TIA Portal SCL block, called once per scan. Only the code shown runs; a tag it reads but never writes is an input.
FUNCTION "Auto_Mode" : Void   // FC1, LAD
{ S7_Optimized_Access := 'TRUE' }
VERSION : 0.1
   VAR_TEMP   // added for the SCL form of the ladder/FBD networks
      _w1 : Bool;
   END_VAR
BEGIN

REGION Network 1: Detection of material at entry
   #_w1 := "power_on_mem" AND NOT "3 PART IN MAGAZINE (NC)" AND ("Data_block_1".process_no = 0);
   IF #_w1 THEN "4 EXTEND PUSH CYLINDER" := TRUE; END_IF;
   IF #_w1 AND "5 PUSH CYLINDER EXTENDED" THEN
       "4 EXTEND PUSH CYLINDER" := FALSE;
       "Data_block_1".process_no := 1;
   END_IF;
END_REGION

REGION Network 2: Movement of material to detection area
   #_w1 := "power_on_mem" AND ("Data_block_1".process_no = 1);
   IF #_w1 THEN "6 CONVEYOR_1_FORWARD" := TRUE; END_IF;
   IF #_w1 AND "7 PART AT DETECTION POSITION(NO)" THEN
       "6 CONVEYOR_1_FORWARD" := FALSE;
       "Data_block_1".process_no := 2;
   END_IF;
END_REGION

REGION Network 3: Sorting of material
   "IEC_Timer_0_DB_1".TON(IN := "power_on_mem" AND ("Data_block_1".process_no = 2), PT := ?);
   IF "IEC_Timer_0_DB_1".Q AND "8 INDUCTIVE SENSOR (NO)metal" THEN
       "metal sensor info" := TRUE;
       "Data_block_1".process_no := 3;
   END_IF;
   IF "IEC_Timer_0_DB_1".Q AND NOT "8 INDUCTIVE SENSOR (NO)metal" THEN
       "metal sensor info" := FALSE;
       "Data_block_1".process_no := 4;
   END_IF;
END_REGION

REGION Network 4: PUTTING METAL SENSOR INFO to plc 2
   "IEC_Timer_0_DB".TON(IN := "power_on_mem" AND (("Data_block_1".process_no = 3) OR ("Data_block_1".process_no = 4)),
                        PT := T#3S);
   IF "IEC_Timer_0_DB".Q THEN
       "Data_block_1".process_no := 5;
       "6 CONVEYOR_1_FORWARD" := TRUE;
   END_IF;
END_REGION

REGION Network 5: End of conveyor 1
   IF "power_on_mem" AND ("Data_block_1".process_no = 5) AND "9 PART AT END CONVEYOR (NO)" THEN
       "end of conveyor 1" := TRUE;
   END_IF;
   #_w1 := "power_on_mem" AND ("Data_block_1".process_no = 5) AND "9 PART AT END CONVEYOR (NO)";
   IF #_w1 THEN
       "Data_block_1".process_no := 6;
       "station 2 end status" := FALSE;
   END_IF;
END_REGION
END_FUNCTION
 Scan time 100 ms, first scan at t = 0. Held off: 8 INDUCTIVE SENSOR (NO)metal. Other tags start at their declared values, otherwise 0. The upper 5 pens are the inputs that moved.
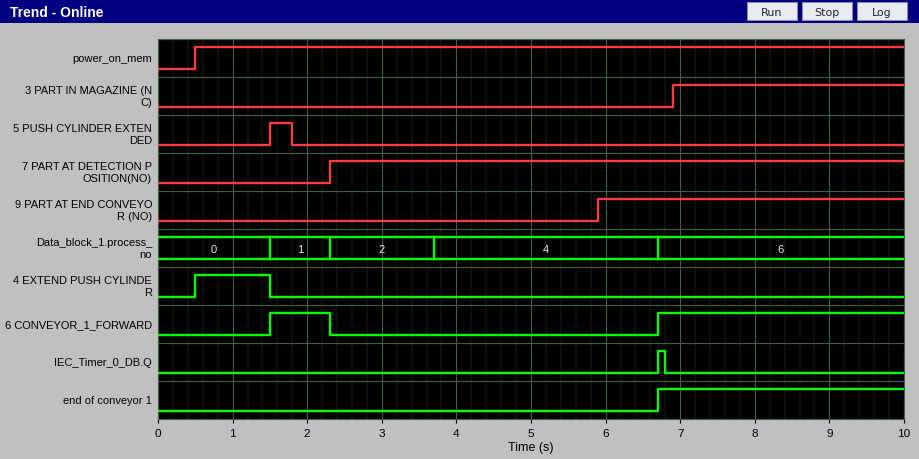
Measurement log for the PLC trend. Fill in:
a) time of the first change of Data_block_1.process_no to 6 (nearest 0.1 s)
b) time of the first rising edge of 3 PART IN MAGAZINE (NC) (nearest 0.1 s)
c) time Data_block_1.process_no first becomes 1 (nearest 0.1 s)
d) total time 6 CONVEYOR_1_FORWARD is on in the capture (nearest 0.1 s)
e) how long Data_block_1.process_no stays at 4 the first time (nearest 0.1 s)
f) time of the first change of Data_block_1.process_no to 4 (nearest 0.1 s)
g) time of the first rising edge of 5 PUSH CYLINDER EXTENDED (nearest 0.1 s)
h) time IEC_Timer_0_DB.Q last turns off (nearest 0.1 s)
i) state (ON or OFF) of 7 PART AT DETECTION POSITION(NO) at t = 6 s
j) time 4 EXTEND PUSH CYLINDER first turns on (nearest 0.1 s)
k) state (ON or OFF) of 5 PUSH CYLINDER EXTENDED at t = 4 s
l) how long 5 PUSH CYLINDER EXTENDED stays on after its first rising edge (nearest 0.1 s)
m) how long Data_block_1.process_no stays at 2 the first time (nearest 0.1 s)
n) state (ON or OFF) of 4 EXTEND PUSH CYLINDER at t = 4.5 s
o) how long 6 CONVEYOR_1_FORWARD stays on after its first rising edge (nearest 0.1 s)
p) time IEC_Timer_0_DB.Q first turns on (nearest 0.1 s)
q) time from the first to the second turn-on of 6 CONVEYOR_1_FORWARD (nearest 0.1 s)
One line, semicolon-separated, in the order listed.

6.7 s; 6.9 s; 1.5 s; 4.1 s; 3.0 s; 3.7 s; 1.5 s; 6.8 s; ON; 0.5 s; OFF; 0.3 s; 1.4 s; OFF; 0.8 s; 6.7 s; 5.2 s
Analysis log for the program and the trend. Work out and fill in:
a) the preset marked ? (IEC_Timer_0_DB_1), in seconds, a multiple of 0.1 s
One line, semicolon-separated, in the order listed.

1.4 s
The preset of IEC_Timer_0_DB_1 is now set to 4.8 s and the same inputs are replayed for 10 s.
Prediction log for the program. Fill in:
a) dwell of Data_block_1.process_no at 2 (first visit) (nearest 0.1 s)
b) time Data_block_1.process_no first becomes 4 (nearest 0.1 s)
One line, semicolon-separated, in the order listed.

4.8 s; 7.1 s
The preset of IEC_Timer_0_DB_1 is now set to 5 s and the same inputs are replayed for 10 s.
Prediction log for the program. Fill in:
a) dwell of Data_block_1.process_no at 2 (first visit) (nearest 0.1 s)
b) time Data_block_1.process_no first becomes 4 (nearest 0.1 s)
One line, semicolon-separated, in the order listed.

5.0 s; 7.3 s
